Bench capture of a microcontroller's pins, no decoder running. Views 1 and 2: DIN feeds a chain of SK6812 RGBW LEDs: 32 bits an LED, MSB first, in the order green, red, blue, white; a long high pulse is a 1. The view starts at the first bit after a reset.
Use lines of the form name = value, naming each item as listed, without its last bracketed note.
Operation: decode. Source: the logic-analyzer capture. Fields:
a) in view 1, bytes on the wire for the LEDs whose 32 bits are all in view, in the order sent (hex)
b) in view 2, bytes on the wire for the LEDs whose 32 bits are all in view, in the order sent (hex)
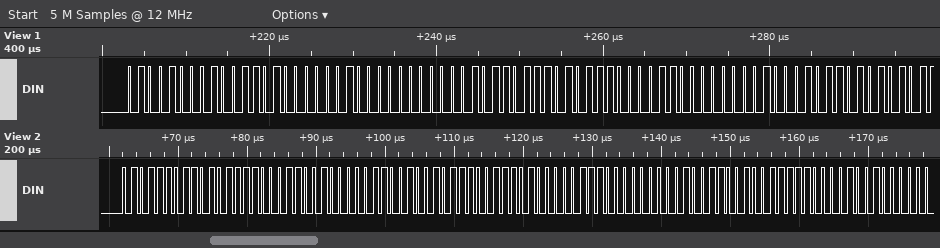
in view 1, bytes on the wire for the LEDs whose 32 bits are all in view, in the order sent = 48 9A 04 00 5B AE 18 04
in view 2, bytes on the wire for the LEDs whose 32 bits are all in view, in the order sent = 5D AF 19 06 4B 9D 07 00
